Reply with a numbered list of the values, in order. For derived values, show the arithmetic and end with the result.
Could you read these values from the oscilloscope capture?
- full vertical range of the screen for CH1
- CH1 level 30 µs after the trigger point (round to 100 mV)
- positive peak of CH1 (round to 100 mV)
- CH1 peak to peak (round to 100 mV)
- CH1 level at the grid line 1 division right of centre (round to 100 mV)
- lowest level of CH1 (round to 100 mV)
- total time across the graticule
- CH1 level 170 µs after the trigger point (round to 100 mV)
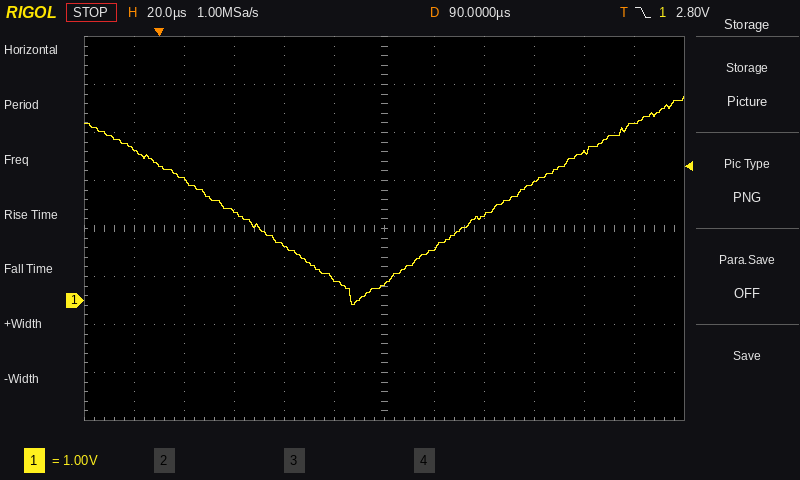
1. 8 V
2. 1.9 V
3. 4.2 V
4. 4.2 V − (-100 mV) = 4.3 V
5. 1.1 V
6. -100 mV
7. 240 µs
8. 3.1 V
